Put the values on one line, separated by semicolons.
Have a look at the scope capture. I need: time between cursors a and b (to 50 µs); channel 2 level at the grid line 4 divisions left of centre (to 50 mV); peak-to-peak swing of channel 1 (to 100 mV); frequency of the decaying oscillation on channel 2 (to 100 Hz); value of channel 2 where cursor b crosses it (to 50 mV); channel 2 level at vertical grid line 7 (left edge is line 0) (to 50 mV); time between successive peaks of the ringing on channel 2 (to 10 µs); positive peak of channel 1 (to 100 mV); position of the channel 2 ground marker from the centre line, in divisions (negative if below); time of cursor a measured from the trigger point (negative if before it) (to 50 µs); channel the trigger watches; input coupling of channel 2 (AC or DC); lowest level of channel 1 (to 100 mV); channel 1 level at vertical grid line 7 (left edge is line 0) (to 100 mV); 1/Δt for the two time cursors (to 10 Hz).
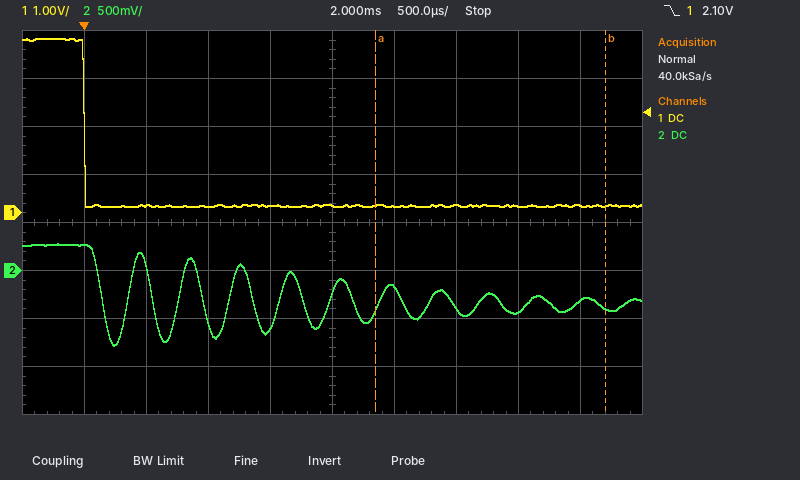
1.85 ms; 250 mV; 3.5 V; 2.5 kHz; -400 mV; -400 mV; 400 µs; 3.6 V; -1.0 div; +2.35 ms; channel 1; DC; 100 mV; 200 mV; 540 Hz
